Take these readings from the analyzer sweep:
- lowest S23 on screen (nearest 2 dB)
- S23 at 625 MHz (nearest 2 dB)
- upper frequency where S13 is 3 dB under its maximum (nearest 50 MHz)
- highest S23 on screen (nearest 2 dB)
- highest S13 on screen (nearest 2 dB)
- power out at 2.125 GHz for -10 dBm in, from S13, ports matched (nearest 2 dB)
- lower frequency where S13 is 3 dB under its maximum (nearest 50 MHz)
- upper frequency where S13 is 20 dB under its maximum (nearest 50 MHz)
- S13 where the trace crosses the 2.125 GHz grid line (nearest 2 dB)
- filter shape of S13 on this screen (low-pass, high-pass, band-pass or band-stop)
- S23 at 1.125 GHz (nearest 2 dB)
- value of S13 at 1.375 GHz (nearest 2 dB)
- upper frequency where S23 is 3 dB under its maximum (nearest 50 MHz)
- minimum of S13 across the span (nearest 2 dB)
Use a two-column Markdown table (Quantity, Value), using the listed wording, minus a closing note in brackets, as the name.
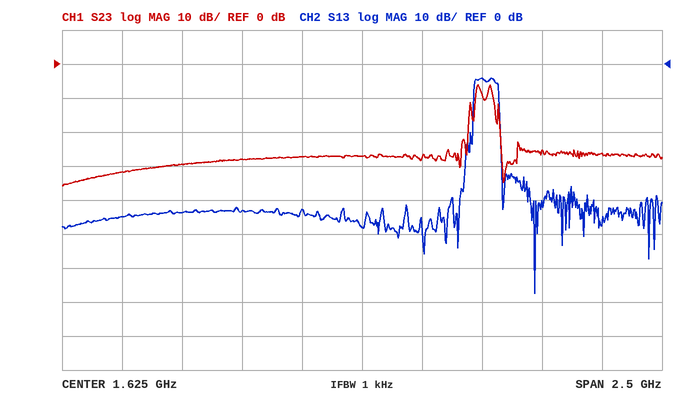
| Quantity | Value |
|---|---|
| lowest S23 on screen | -36 dB |
| S23 at 625 MHz | -32 dB |
| upper frequency where S13 is 3 dB under its maximum | 2.20 GHz |
| highest S23 on screen | -6 dB |
| highest S13 on screen | -4 dB |
| power out at 2.125 GHz for -10 dBm in, from S13, ports matched | -14 dBm |
| lower frequency where S13 is 3 dB under its maximum | 2.10 GHz |
| upper frequency where S13 is 20 dB under its maximum | 2.20 GHz |
| S13 where the trace crosses the 2.125 GHz grid line | -4 dB |
| filter shape of S13 on this screen | band-pass |
| S23 at 1.125 GHz | -28 dB |
| value of S13 at 1.375 GHz | -42 dB |
| upper frequency where S23 is 3 dB under its maximum | 2.15 GHz |
| minimum of S13 across the span | -68 dB |
